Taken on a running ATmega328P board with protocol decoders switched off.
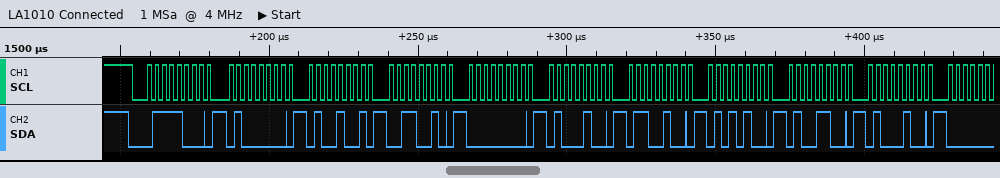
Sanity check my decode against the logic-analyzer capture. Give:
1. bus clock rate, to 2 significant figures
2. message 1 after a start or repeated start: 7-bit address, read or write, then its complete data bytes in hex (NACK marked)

400 kHz
0x3C write: 40 49 32 00 44 64 54 4C 44
